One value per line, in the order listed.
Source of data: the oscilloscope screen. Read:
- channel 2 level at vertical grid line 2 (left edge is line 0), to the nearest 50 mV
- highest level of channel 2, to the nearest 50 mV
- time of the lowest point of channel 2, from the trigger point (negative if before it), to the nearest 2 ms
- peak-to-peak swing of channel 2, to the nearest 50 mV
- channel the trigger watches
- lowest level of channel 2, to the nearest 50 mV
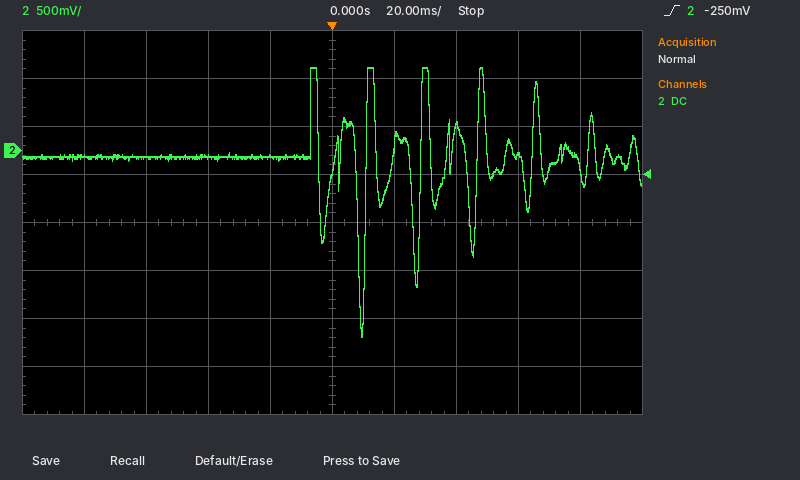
-50 mV
850 mV
+10 ms
2.80 V
channel 2
-1.95 V
